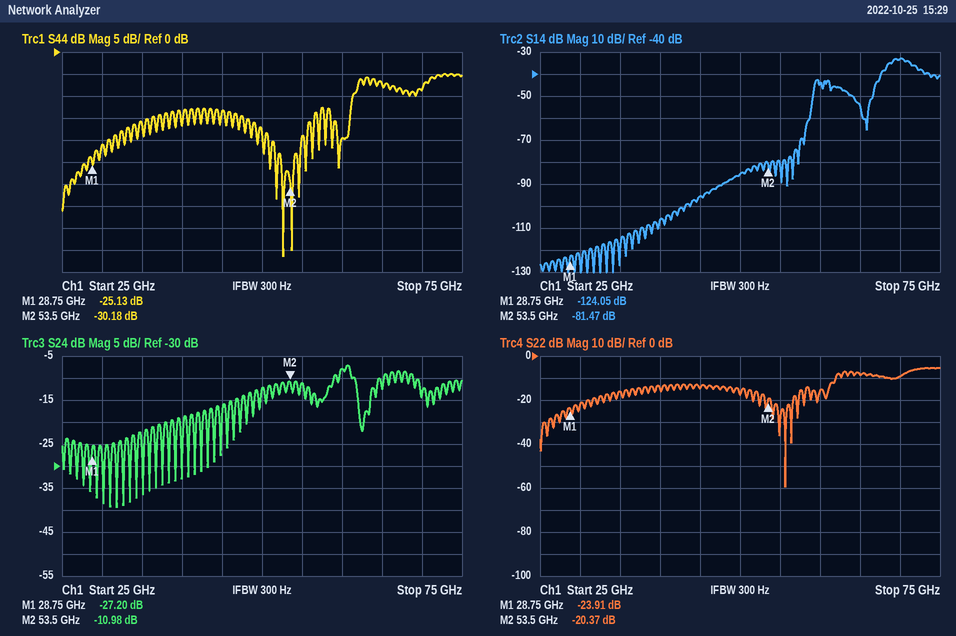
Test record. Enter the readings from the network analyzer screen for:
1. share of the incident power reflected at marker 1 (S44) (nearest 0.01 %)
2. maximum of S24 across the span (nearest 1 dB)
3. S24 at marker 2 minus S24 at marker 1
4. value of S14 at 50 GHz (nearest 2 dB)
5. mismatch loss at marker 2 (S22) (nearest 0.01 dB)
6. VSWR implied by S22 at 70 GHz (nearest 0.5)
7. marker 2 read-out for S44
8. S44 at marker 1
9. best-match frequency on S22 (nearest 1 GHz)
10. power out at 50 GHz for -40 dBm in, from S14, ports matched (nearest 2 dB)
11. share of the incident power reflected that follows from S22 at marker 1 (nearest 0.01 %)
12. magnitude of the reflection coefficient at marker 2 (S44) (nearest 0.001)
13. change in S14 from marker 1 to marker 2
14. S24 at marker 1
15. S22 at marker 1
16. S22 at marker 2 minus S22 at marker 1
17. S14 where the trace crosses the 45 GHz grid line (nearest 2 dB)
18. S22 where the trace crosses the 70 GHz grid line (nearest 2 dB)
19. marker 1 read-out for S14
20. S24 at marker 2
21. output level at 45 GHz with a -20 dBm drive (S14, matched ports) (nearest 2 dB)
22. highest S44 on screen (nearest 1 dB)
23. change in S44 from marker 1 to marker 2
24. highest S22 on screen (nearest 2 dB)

0.31 %
-7 dB
16.22 dB
-86 dB
0.04 dB
2.0
-30.18 dB
-25.13 dB
56 GHz
-126 dBm
0.41 %
0.031
42.58 dB
-27.20 dB
-23.91 dB
3.54 dB
-96 dB
-10 dB
-124.05 dB
-10.98 dB
-116 dBm
-5 dB
-5.05 dB
-6 dB
